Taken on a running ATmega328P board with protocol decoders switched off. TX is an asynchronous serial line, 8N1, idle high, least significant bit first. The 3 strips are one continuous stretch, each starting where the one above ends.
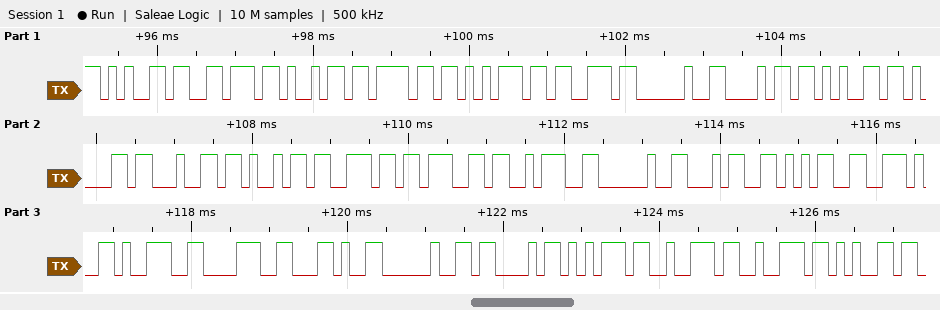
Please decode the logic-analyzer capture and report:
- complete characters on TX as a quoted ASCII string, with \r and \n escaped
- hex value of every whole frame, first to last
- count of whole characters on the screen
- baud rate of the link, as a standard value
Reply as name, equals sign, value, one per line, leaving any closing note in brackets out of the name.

complete characters on TX as a quoted ASCII string, with \r and \n escaped = "evious heading: 45.98, Curre"
hex value of every whole frame, first to last = 65 76 69 6F 75 73 20 68 65 61 64 69 6E 67 3A 20 34 35 2E 39 38 2C 20 43 75 72 72 65
count of whole characters on the screen = 28
baud rate of the link, as a standard value = 9600 baud
